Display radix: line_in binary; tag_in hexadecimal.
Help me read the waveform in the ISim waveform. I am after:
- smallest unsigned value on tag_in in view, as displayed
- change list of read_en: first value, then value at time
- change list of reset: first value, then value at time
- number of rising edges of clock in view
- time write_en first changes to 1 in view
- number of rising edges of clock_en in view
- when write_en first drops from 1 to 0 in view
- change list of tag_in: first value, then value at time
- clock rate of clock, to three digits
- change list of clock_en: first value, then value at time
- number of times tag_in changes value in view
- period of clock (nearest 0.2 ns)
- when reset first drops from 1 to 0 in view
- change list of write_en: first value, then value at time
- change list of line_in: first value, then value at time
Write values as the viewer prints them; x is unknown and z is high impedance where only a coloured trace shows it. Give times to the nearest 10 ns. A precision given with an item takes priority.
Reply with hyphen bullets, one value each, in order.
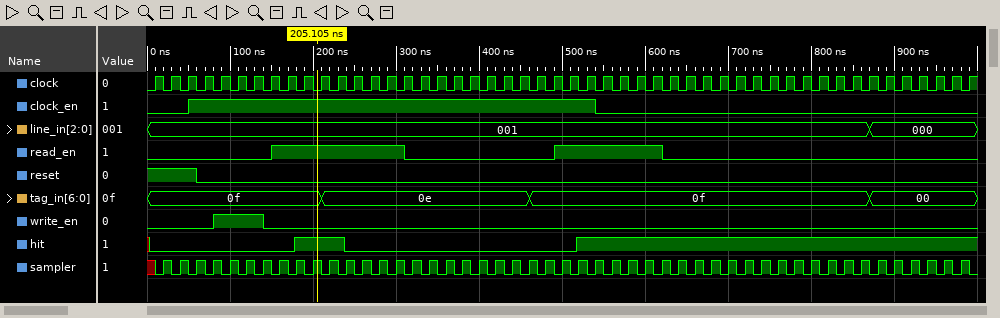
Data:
- 00
- 0, 1 at 150 ns, 0 at 310 ns, 1 at 490 ns, 0 at 620 ns
- 1, 0 at 60 ns
- 50
- 80 ns
- 1
- 140 ns
- 0f, 0e at 210 ns, 0f at 460 ns, 00 at 870 ns
- 50.0 MHz
- 0, 1 at 50 ns, 0 at 540 ns
- 3
- 20 ns
- 60 ns
- 0, 1 at 80 ns, 0 at 140 ns
- 001, 000 at 870 ns
